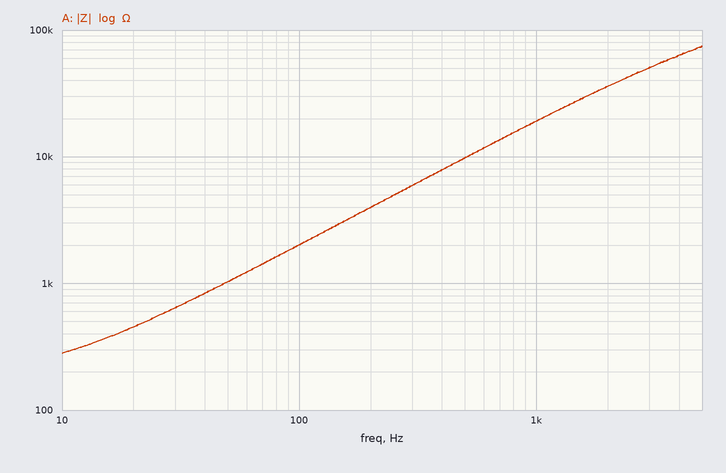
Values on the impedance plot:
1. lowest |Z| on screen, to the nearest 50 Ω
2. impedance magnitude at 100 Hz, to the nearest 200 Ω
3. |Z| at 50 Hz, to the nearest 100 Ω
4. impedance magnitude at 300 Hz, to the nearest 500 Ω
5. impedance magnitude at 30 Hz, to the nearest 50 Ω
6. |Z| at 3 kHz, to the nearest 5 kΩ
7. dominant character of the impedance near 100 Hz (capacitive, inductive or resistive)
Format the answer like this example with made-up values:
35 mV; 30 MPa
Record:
300 Ω; 2.0 kΩ; 1.0 kΩ; 6.0 kΩ; 650 Ω; 50 kΩ; inductive
